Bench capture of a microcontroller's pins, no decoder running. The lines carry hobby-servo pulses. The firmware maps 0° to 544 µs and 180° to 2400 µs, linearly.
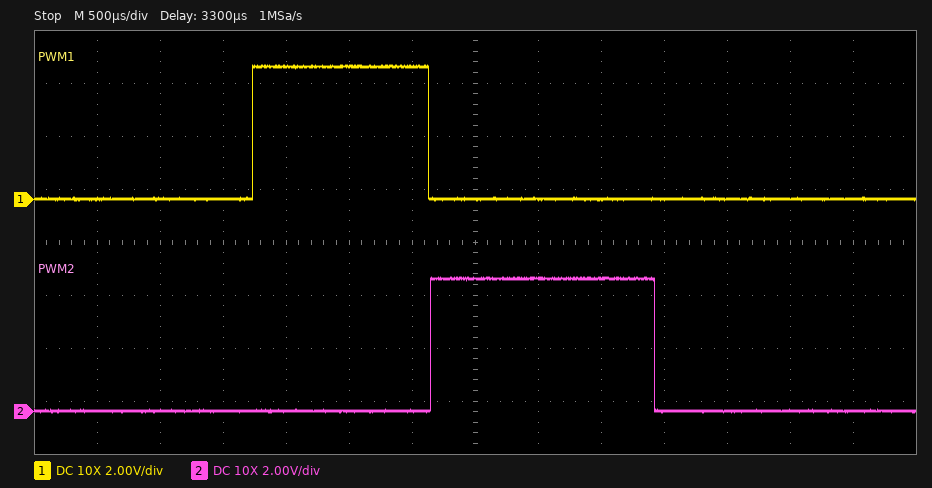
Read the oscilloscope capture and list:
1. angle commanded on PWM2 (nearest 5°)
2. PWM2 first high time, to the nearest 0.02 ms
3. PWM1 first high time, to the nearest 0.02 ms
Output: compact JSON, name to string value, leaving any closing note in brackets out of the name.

{"angle commanded on PWM2": "120°", "PWM2 first high time, to the nearest 0.02 ms": "1.78 ms", "PWM1 first high time, to the nearest 0.02 ms": "1.40 ms"}
